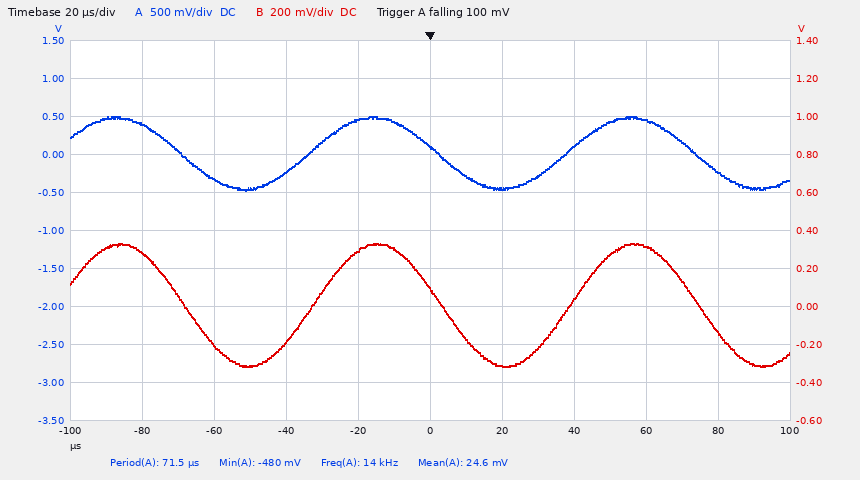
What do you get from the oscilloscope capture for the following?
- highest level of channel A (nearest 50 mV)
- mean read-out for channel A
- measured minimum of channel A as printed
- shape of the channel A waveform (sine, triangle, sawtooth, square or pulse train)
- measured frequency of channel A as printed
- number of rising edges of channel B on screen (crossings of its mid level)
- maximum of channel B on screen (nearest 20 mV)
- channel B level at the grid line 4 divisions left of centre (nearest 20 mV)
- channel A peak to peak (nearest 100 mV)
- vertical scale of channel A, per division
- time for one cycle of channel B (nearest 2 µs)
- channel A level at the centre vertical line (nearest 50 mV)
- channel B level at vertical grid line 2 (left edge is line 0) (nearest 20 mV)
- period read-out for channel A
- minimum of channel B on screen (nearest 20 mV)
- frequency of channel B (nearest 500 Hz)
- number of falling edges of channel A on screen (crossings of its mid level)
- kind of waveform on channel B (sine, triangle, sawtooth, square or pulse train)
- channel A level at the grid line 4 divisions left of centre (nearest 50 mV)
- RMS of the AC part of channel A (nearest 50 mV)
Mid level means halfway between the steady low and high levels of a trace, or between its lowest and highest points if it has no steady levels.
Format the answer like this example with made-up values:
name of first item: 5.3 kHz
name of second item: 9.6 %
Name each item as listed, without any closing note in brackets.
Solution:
highest level of channel A: 500 mV
mean read-out for channel A: 24.6 mV
measured minimum of channel A as printed: -480 mV
shape of the channel A waveform: sine
measured frequency of channel A as printed: 14 kHz
number of rising edges of channel B on screen: 2
maximum of channel B on screen: 340 mV
channel B level at the grid line 4 divisions left of centre: 280 mV
channel A peak to peak: 1.00 V
vertical scale of channel A, per division: 500 mV
time for one cycle of channel B: 72 µs
channel A level at the centre vertical line: 100 mV
channel B level at vertical grid line 2 (left edge is line 0): -200 mV
period read-out for channel A: 71.5 µs
minimum of channel B on screen: -320 mV
frequency of channel B: 14.0 kHz
number of falling edges of channel A on screen: 3
kind of waveform on channel B: sine
channel A level at the grid line 4 divisions left of centre: 400 mV
RMS of the AC part of channel A: 350 mV
